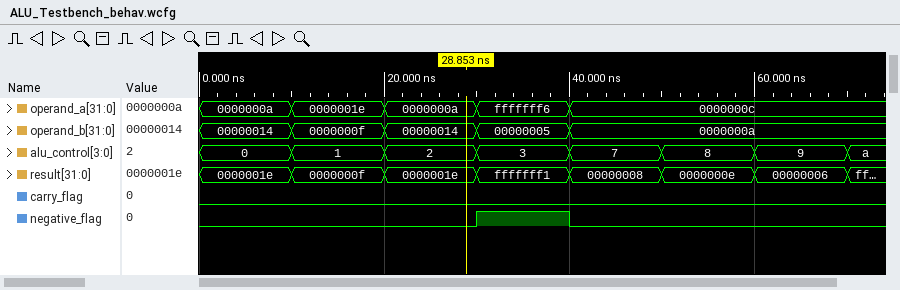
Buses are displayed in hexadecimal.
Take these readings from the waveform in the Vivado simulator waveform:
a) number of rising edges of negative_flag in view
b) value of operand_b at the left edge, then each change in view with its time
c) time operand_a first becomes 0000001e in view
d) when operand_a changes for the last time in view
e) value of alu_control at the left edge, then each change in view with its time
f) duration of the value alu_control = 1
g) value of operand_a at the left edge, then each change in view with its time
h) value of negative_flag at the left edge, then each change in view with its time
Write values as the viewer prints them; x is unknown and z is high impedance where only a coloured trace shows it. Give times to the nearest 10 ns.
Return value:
1
00000014, 0000000f at 10 ns, 00000014 at 20 ns, 00000005 at 30 ns, 0000000a at 40 ns
10 ns
40 ns
0, 1 at 10 ns, 2 at 20 ns, 3 at 30 ns, 7 at 40 ns, 8 at 50 ns, 9 at 60 ns, a at 70 ns
10 ns
0000000a, 0000001e at 10 ns, 0000000a at 20 ns, fffffff6 at 30 ns, 0000000c at 40 ns
0, 1 at 30 ns, 0 at 40 ns
